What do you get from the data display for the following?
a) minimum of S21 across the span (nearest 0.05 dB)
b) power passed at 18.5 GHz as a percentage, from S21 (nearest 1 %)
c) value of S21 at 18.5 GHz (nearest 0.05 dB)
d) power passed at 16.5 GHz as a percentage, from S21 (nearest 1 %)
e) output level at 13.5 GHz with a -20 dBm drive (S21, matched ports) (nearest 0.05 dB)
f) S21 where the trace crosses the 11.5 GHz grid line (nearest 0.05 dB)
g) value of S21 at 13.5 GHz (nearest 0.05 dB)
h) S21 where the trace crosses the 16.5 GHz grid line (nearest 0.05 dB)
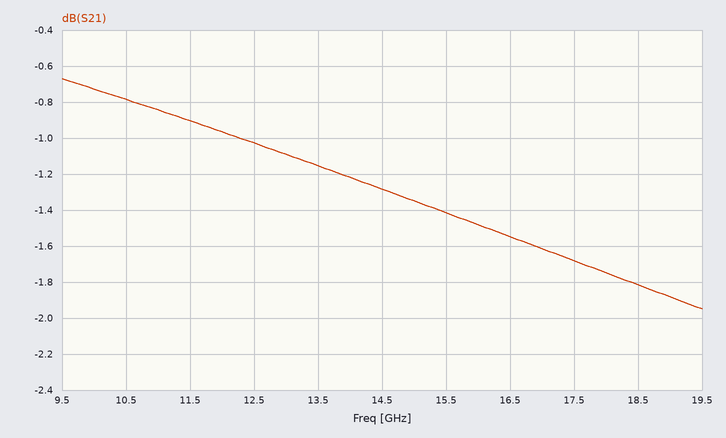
-1.95 dB
66 %
-1.80 dB
70 %
-21.15 dBm
-0.90 dB
-1.15 dB
-1.55 dB
